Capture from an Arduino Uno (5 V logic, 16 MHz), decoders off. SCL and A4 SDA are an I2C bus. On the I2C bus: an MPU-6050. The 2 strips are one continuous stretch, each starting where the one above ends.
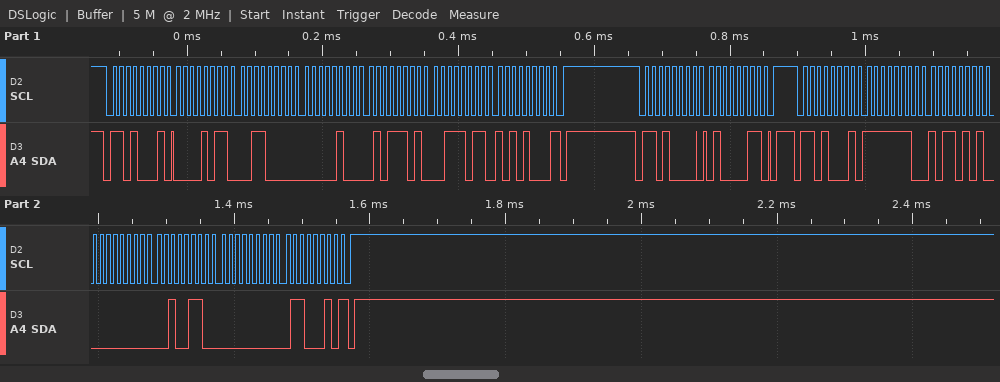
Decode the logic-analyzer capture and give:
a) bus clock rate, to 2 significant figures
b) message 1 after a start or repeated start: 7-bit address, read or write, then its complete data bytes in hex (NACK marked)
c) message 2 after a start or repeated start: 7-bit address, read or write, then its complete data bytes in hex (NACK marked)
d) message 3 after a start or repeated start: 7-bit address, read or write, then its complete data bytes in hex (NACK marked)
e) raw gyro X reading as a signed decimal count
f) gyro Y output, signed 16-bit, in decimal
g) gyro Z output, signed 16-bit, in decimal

100 kHz
0x68 read: 0B 30 04 5D 3B A8 NACK
0x68 write: 43
0x68 read: FE B5 00 26 00 62 NACK
-331
38
98
